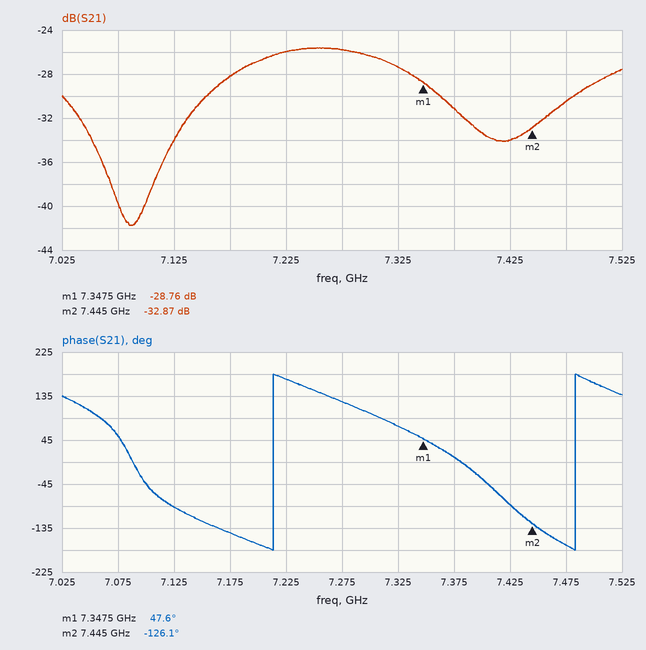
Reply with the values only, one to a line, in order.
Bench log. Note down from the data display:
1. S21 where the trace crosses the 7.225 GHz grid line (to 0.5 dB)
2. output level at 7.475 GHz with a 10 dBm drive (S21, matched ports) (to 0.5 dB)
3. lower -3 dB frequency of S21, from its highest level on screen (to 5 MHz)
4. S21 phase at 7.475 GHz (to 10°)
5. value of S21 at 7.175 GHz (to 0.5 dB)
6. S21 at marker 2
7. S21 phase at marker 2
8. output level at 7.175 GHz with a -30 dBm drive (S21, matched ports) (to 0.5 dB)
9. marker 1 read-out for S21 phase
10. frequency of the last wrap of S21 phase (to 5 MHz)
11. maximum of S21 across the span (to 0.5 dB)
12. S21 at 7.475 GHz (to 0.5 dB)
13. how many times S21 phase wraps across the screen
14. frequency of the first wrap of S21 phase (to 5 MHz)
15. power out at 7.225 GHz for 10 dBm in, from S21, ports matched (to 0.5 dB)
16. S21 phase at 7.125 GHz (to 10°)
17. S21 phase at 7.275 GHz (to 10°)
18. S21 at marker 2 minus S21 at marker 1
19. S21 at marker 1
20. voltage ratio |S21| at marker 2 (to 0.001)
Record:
-26.0 dB
-20.5 dBm
7.170 GHz
-170°
-28.0 dB
-32.87 dB
-126.1°
-58.0 dBm
47.6°
7.485 GHz
-25.5 dB
-30.5 dB
2
7.215 GHz
-16.0 dBm
-90°
120°
-4.11 dB
-28.76 dB
0.023
